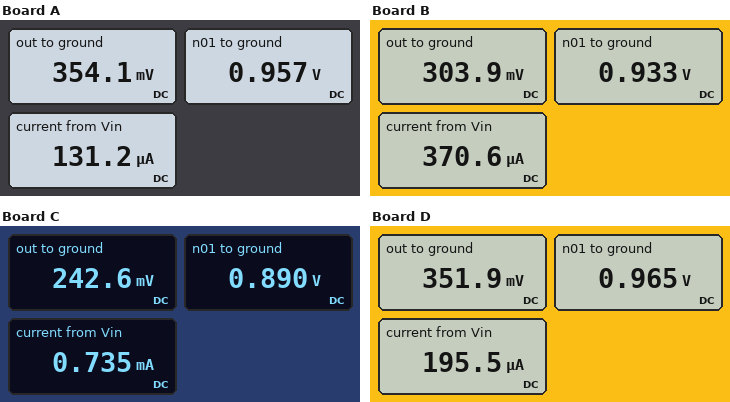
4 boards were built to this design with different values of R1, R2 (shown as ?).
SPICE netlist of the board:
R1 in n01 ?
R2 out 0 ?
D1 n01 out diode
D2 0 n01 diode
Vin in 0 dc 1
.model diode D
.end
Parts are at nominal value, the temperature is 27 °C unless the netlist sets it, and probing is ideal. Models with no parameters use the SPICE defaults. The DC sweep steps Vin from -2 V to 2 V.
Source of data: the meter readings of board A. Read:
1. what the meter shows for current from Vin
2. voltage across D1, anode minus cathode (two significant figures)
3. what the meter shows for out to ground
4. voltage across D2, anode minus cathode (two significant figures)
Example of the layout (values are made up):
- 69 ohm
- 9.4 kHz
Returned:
- 131.2 µA
- 600 mV
- 354.1 mV
- -960 mV
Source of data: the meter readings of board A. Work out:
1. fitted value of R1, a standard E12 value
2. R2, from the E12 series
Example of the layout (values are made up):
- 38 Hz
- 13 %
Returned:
- 330 Ω
- 2.7 kΩ
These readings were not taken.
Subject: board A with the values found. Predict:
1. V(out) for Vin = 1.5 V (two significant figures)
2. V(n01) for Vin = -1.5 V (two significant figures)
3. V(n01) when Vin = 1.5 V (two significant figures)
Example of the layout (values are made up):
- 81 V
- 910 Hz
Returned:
- 780 mV
- -680 mV
- 1.4 V
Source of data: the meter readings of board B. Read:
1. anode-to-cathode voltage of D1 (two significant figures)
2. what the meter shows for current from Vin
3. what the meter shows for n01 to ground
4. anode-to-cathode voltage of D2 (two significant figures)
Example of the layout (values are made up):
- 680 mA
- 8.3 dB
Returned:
- 630 mV
- 370.6 µA
- 0.933 V
- -930 mV
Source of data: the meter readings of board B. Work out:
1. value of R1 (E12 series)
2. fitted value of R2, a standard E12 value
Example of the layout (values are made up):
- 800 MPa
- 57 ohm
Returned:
- 180 Ω
- 820 Ω
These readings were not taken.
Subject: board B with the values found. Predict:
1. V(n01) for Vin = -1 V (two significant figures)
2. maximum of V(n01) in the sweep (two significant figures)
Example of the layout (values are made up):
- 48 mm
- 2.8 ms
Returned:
- -670 mV
- 1.8 V
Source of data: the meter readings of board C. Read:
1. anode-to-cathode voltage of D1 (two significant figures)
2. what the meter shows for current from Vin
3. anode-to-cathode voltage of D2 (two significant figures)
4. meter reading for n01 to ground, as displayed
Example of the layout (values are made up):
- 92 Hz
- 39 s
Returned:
- 650 mV
- 0.735 mA
- -890 mV
- 0.890 V
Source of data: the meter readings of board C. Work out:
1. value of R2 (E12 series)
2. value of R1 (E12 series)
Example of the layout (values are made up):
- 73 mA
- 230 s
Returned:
- 330 Ω
- 150 Ω
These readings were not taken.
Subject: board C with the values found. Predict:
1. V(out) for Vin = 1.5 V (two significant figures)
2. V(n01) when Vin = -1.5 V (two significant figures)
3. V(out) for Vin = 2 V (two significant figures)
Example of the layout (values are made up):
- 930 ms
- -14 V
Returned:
- 570 mV
- -700 mV
- 910 mV
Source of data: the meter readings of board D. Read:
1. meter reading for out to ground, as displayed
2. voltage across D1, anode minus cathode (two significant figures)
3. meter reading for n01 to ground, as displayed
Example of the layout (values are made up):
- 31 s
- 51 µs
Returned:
- 351.9 mV
- 610 mV
- 0.965 V
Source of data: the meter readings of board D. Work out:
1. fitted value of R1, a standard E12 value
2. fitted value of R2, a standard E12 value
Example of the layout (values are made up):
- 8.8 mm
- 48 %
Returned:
- 180 Ω
- 1.8 kΩ
